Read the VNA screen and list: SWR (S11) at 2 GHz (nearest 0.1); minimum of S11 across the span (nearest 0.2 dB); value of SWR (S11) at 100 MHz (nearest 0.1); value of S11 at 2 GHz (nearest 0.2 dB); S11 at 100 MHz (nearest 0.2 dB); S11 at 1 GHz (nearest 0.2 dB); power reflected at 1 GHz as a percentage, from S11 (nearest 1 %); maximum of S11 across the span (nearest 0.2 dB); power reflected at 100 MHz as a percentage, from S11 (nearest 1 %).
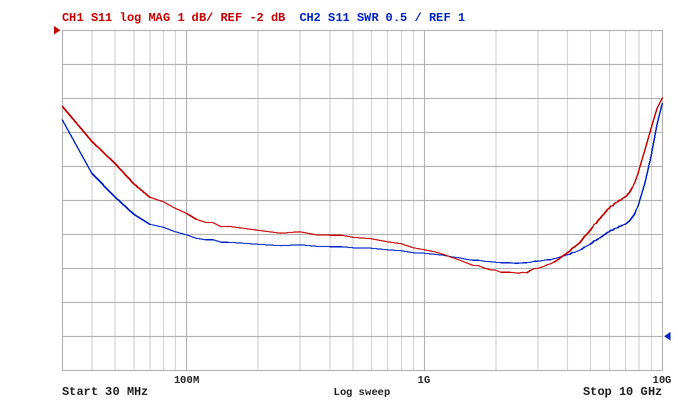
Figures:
2.1
-9.2 dB
2.5
-9.0 dB
-7.4 dB
-8.4 dB
14 %
-4.0 dB
18 %
